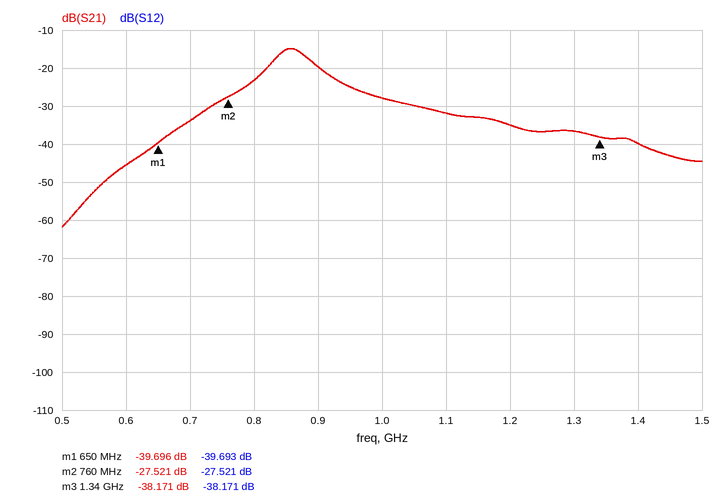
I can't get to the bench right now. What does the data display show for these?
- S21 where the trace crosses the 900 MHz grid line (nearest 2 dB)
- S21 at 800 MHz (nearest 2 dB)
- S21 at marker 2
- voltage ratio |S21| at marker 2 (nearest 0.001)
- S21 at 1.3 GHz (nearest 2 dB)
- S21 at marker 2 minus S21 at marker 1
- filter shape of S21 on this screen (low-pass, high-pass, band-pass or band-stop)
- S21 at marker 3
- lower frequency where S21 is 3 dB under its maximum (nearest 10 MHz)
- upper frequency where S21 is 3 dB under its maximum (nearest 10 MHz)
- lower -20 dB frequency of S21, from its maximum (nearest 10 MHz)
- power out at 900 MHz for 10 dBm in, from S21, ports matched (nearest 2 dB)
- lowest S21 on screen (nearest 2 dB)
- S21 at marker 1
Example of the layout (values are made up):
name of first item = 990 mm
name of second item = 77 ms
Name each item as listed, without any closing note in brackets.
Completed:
S21 where the trace crosses the 900 MHz grid line = -20 dB
S21 at 800 MHz = -24 dB
S21 at marker 2 = -27.521 dB
voltage ratio |S21| at marker 2 = 0.042
S21 at 1.3 GHz = -36 dB
S21 at marker 2 minus S21 at marker 1 = 12.175 dB
filter shape of S21 on this screen = band-pass
S21 at marker 3 = -38.171 dB
lower frequency where S21 is 3 dB under its maximum = 830 MHz
upper frequency where S21 is 3 dB under its maximum = 890 MHz
lower -20 dB frequency of S21, from its maximum = 690 MHz
power out at 900 MHz for 10 dBm in, from S21, ports matched = -10 dBm
lowest S21 on screen = -62 dB
S21 at marker 1 = -39.696 dB
